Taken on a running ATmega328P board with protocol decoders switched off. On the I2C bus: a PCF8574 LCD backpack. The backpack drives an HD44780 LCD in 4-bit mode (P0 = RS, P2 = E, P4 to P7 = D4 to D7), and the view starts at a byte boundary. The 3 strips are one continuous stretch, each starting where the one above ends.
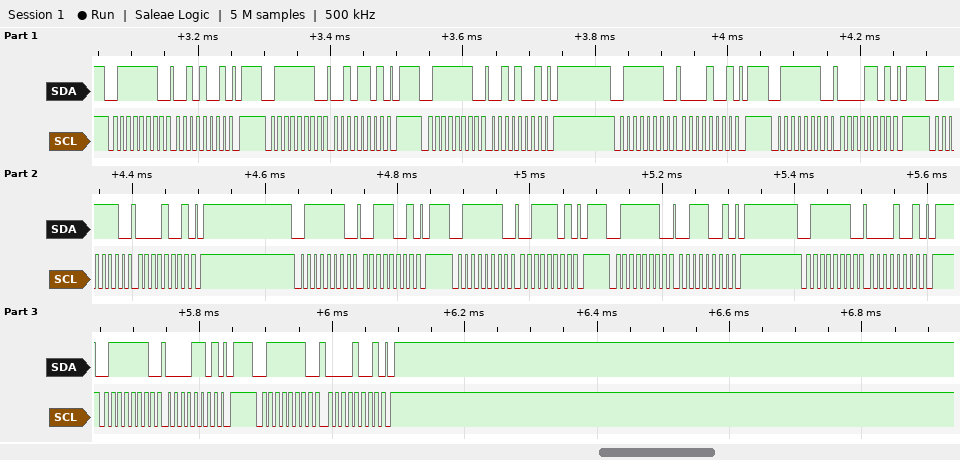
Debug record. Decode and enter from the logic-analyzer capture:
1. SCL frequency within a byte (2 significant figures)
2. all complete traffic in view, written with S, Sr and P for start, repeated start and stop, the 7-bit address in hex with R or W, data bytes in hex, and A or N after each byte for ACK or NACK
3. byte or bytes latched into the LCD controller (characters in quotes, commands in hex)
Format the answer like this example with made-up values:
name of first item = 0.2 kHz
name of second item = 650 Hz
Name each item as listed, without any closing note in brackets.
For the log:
SCL frequency within a byte = 100 kHz
all complete traffic in view, written with S, Sr and P for start, repeated start and stop, the 7-bit address in hex with R or W, data bytes in hex, and A or N after each byte for ACK or NACK = S 3FW A 29 A P S 3FW A 2D A P S 3FW A 29 A P S 3FW A 09 A P S 3FW A 0D A P S 3FW A 09 A P S 3FW A 39 A P S 3FW A 3D A P S 3FW A 39 A P S 3FW A 09 A P S 3FW A 0D A P S 3FW A 09 A P
byte or bytes latched into the LCD controller = ' ' '0'
